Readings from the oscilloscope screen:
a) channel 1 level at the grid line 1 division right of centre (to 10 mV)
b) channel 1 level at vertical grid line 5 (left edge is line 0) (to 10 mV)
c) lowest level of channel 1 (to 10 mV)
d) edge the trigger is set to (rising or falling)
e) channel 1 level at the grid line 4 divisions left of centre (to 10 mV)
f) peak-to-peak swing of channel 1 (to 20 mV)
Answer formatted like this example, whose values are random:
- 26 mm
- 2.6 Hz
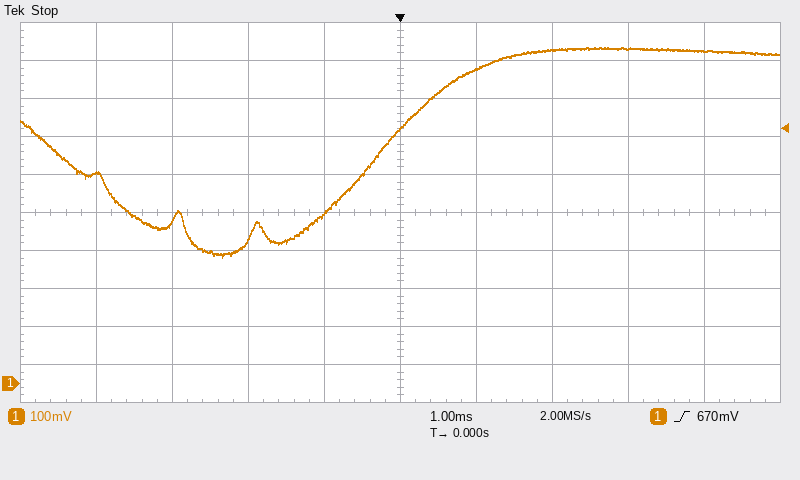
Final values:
- 830 mV
- 670 mV
- 330 mV
- rising
- 550 mV
- 560 mV
